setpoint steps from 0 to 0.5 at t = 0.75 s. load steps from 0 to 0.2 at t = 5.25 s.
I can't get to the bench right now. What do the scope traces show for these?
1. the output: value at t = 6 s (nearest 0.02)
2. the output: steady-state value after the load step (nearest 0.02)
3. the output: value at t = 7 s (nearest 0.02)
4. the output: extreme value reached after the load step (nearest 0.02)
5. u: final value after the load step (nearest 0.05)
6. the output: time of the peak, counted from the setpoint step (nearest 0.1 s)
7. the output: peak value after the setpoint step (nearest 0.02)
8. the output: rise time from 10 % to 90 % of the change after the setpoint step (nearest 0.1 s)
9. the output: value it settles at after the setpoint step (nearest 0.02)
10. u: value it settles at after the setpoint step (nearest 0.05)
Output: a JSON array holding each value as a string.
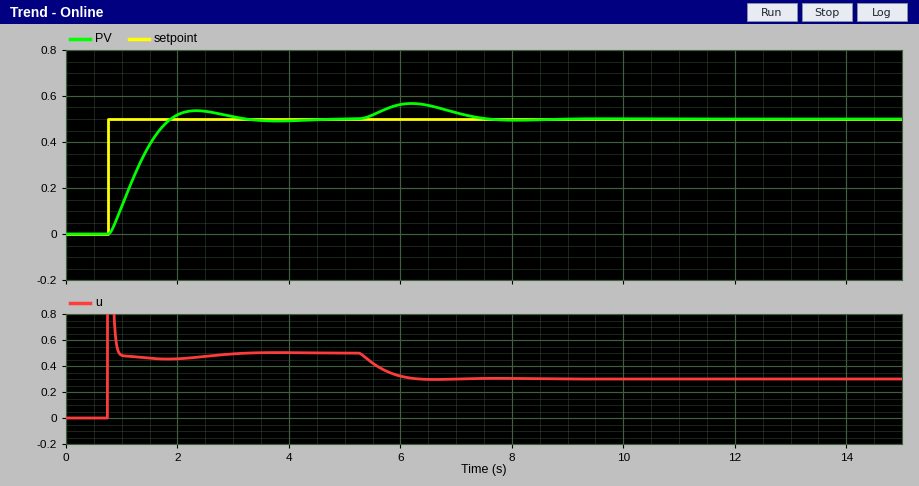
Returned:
["0.56", "0.50", "0.52", "0.56", "0.30", "1.6 s", "0.54", "0.8 s", "0.50", "0.50"]
